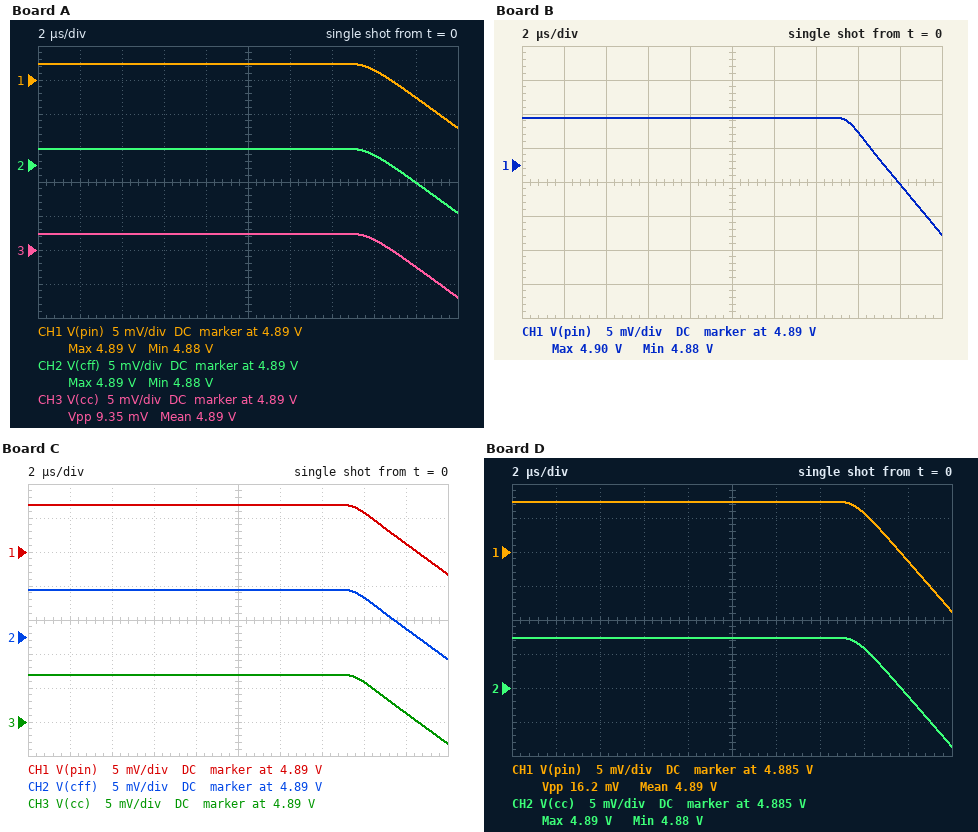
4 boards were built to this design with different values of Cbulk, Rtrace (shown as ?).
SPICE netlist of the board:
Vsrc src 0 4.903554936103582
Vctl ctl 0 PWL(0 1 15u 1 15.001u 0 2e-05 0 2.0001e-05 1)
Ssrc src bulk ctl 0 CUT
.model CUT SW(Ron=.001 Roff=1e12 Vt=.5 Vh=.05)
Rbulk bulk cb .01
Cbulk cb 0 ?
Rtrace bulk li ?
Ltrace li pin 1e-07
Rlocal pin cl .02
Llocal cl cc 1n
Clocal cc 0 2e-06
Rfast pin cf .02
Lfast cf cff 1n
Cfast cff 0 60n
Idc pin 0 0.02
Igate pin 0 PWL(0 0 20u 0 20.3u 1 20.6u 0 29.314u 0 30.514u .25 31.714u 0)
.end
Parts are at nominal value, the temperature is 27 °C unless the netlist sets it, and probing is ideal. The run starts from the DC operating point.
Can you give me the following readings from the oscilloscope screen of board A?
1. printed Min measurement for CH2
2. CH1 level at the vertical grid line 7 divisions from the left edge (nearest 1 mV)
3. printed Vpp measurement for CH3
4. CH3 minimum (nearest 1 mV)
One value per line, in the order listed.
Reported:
4.88 V
4.892 V
9.35 mV
4.883 V
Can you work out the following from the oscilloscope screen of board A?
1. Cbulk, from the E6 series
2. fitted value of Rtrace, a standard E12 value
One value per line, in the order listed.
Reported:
6.8 µF
0.56 Ω
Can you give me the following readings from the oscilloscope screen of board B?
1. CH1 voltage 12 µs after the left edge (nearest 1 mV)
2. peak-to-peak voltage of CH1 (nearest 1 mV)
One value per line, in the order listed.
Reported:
4.897 V
17 mV
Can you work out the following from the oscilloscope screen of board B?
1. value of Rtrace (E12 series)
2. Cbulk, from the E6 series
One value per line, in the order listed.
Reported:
0.33 Ω
3.3 µF
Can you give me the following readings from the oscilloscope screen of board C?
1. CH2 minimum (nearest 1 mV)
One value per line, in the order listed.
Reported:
4.887 V
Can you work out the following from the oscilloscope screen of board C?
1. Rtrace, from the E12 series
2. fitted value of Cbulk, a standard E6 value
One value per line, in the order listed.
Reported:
0.33 Ω
6.8 µF
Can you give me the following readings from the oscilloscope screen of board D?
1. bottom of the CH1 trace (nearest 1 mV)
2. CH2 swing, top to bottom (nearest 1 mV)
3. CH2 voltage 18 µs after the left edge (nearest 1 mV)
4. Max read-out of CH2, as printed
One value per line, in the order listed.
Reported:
4.876 V
16 mV
4.884 V
4.89 V
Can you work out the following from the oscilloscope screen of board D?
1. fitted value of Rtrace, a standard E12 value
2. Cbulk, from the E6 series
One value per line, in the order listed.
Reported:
0.56 Ω
3.3 µF
